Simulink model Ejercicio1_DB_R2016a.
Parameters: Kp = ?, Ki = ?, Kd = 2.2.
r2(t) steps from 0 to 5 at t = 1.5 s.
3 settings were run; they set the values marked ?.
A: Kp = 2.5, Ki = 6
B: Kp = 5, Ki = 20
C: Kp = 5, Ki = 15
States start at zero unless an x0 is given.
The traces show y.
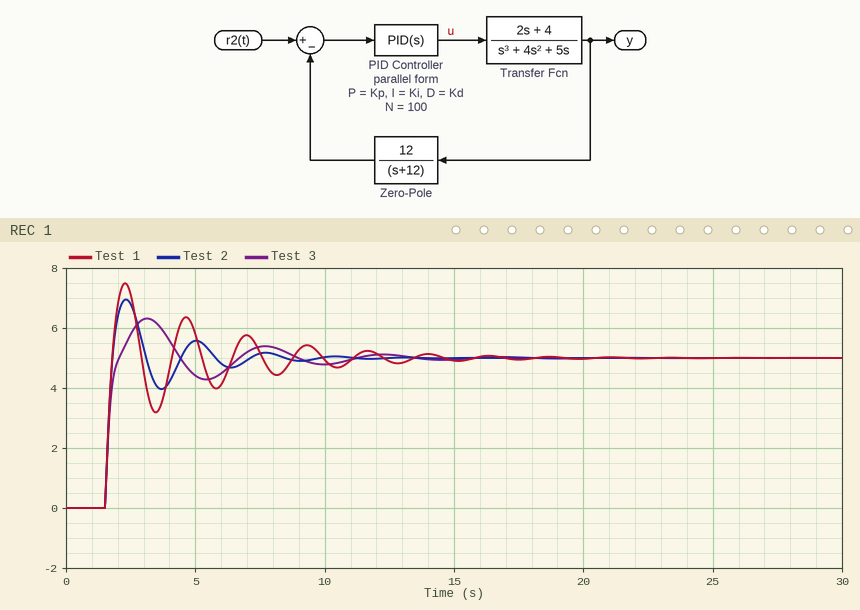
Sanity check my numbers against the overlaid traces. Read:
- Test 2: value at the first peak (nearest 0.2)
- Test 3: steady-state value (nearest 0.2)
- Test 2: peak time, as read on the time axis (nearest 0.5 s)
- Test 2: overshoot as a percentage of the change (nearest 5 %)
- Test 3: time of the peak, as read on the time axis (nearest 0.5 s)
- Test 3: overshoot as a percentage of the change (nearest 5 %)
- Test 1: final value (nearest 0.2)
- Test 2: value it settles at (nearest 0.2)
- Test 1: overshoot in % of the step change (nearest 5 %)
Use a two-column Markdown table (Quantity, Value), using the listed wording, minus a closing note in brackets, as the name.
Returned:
| Quantity | Value |
|---|---|
| Test 2: value at the first peak | 7.0 |
| Test 3: steady-state value | 5.0 |
| Test 2: peak time, as read on the time axis | 2.5 s |
| Test 2: overshoot as a percentage of the change | 40 % |
| Test 3: time of the peak, as read on the time axis | 3.0 s |
| Test 3: overshoot as a percentage of the change | 25 % |
| Test 1: final value | 5.0 |
| Test 2: value it settles at | 5.0 |
| Test 1: overshoot in % of the step change | 50 % |
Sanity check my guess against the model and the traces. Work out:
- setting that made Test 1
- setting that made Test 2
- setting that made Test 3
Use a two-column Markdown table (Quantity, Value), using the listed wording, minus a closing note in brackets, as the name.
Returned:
| Quantity | Value |
|---|---|
| setting that made Test 1 | B |
| setting that made Test 2 | C |
| setting that made Test 3 | A |
